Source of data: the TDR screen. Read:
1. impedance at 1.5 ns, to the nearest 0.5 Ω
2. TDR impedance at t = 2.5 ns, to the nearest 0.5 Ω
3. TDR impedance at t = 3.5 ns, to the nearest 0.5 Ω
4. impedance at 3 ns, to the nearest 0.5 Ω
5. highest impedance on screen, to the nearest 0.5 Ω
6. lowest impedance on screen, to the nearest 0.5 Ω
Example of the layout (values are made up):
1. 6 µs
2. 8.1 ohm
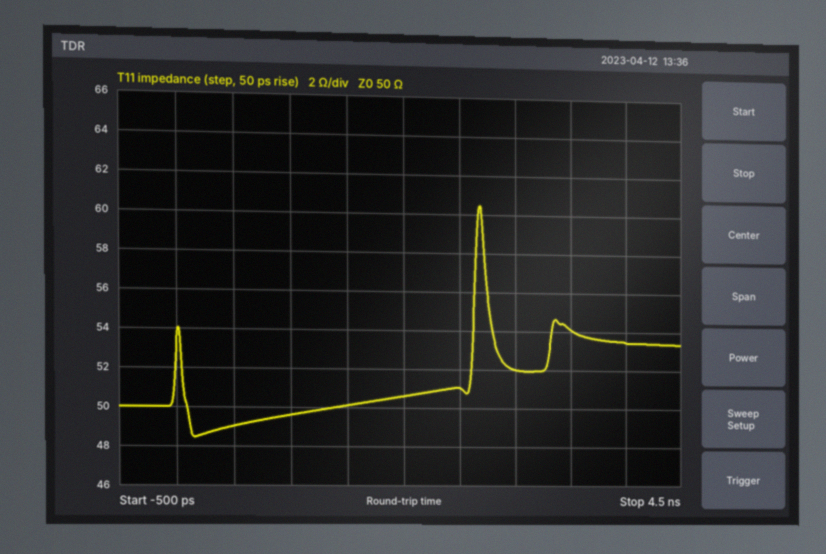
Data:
1. 50.0 Ω
2. 51.0 Ω
3. 54.0 Ω
4. 52.0 Ω
5. 60.5 Ω
6. 48.5 Ω
